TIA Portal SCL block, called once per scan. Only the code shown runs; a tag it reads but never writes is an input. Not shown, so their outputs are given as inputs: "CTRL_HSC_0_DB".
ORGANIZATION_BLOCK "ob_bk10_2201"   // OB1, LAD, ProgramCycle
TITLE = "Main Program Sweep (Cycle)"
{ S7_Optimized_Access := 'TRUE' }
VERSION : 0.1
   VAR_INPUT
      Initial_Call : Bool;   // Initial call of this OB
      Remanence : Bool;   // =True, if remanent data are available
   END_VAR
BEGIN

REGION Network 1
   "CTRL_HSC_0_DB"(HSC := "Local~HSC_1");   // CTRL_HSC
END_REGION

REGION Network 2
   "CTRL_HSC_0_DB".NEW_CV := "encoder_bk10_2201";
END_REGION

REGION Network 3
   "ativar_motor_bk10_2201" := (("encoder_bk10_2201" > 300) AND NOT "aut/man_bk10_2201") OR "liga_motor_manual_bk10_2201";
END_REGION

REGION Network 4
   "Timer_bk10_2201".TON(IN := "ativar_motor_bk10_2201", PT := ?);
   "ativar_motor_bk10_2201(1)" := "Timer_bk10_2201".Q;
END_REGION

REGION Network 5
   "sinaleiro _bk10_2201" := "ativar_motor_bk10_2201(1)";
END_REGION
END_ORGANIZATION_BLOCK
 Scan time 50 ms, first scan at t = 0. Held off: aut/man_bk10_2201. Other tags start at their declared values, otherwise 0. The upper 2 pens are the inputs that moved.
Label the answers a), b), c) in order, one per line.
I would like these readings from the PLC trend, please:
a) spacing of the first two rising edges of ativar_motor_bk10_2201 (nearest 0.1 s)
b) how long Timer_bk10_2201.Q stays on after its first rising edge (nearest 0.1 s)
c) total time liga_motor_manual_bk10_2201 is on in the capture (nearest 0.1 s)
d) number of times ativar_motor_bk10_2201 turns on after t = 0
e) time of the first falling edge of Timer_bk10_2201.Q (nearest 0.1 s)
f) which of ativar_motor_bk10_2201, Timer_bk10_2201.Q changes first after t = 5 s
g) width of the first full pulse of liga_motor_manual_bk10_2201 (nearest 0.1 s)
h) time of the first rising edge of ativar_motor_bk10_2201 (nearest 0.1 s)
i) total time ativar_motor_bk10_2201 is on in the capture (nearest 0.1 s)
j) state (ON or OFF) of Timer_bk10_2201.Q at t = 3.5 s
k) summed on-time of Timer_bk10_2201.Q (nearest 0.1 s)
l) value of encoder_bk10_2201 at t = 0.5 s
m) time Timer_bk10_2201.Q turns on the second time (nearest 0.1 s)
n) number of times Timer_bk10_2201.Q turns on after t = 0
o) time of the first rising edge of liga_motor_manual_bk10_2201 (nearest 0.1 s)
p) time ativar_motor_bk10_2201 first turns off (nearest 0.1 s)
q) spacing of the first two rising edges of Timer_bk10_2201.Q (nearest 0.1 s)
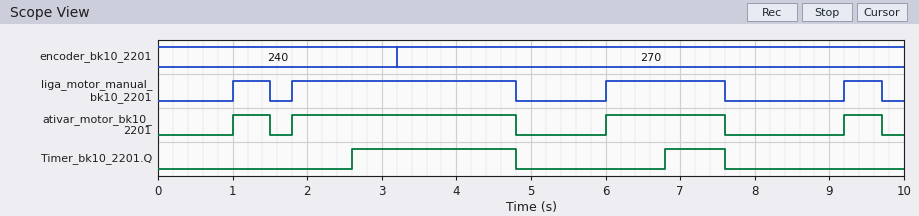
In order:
a) 0.8 s
b) 2.2 s
c) 5.6 s
d) 4
e) 4.8 s
f) ativar_motor_bk10_2201
g) 0.5 s
h) 1.0 s
i) 5.6 s
j) ON
k) 3.0 s
l) 240
m) 6.8 s
n) 2
o) 1.0 s
p) 1.5 s
q) 4.2 s
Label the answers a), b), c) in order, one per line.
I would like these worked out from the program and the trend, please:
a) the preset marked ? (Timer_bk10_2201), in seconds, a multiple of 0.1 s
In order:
a) 0.8 s
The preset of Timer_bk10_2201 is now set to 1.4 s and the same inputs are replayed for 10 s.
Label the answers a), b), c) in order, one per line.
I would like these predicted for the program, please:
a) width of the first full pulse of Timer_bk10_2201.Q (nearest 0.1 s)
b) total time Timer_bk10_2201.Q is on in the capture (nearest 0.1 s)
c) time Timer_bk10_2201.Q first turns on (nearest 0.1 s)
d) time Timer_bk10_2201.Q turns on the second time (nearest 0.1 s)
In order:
a) 1.6 s
b) 1.8 s
c) 3.2 s
d) 7.4 s
